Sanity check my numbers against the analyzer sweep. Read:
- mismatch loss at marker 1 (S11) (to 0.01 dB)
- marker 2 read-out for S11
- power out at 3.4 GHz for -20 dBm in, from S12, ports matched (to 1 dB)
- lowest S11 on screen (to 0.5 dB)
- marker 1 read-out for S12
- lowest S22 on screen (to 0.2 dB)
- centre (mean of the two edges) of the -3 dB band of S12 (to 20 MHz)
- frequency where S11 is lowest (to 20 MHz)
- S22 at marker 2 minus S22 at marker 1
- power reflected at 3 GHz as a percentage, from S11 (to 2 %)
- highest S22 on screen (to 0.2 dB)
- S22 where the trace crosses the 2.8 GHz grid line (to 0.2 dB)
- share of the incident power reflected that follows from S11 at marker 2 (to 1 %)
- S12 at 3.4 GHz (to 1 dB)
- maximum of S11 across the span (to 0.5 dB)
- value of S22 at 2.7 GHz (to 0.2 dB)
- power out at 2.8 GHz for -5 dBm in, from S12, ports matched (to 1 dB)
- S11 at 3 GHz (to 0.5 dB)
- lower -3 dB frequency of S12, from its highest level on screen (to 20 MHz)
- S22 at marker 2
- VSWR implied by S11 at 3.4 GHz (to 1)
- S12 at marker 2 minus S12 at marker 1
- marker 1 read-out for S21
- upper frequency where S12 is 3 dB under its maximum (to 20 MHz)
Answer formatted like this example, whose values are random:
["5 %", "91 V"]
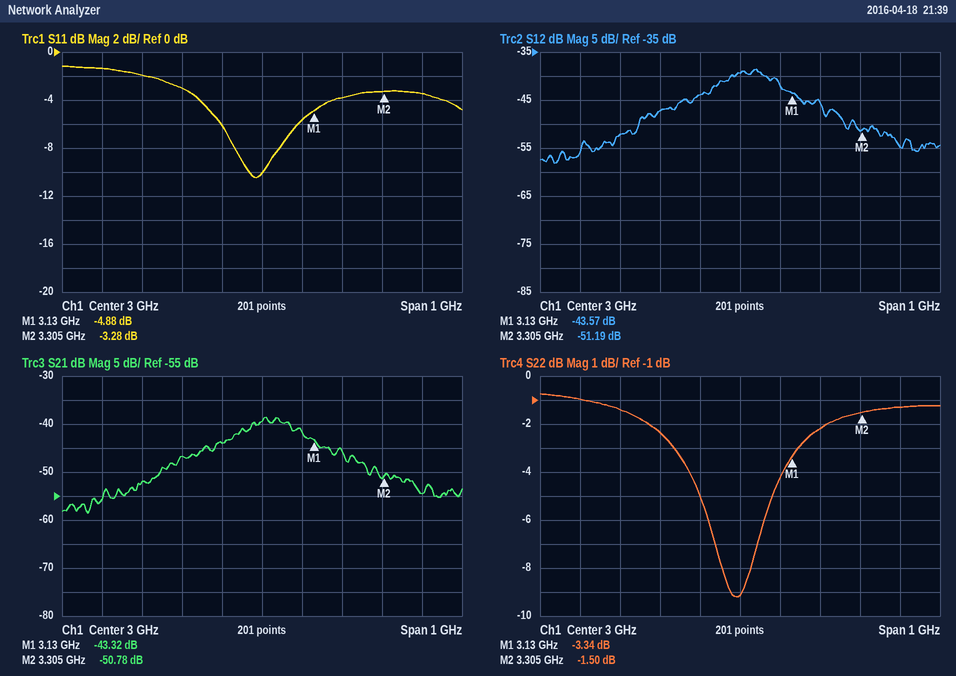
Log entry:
["1.71 dB", "-3.28 dB", "-75 dBm", "-10.5 dB", "-43.57 dB", "-9.2 dB", "3.02 GHz", "2.98 GHz", "1.84 dB", "10 %", "-0.8 dB", "-2.4 dB", "47 %", "-55 dB", "-1.0 dB", "-1.4 dB", "-52 dBm", "-10.0 dB", "2.94 GHz", "-1.50 dB", "5", "-7.62 dB", "-43.32 dB", "3.10 GHz"]
